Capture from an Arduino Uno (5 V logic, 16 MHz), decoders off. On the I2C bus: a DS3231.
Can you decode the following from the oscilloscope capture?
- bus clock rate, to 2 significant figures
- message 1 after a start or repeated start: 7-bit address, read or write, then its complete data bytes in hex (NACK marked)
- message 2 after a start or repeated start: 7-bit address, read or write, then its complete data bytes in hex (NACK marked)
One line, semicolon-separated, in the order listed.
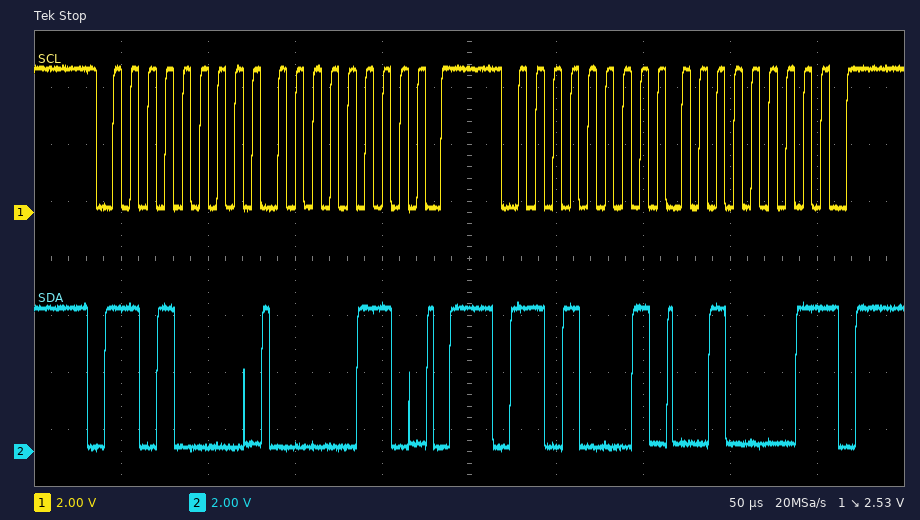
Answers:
100 kHz; 0x68 write: 06; 0x68 read: 21 NACK
